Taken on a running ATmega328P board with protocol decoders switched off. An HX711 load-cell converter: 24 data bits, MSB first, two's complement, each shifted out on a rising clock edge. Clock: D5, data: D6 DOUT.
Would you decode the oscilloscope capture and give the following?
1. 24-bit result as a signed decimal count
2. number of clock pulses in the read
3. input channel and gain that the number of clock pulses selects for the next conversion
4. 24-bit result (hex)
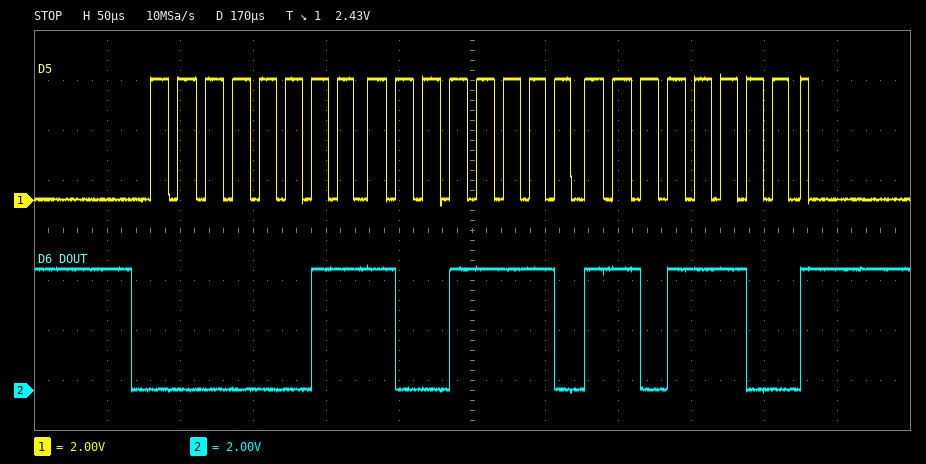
237276
25
channel A, gain 128
0x039EDC
